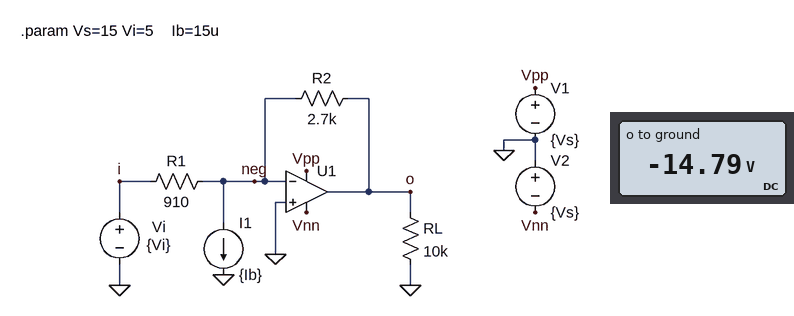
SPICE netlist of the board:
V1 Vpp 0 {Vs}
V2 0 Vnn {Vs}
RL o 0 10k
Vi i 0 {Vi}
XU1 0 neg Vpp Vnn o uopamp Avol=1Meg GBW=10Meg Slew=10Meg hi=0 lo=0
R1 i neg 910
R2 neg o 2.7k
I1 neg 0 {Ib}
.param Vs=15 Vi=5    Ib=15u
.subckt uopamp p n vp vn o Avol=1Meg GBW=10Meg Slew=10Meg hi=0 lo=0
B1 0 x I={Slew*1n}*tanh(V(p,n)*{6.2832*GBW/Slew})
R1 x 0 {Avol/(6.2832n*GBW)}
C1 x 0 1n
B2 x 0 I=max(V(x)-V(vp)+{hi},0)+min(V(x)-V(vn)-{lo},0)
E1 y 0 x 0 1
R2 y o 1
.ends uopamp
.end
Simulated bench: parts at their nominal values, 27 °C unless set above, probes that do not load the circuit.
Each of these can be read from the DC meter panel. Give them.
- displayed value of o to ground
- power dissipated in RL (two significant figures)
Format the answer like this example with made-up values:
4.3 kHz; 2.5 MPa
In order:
-14.79 V; 22 mW
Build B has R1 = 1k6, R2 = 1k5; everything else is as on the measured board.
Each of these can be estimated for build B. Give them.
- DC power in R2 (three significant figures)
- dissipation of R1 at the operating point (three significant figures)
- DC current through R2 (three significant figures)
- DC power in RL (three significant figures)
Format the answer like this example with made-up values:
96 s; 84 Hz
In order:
14.5 mW; 15.6 mW; 3.11 mA; 2.18 mW
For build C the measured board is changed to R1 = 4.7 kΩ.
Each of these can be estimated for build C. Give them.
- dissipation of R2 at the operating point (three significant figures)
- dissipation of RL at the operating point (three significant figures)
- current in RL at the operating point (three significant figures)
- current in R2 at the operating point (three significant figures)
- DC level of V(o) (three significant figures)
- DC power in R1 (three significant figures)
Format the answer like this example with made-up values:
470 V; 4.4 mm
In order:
2.97 mW; 802 µW; 283 µA; 1.05 mA; -2.83 V; 5.32 mW
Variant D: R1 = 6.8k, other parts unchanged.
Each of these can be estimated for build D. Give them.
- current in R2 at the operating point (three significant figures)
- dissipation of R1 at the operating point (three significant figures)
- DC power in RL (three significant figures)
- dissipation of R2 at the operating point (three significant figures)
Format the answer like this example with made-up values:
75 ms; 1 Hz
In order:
720 µA; 3.68 mW; 378 µW; 1.40 mW
